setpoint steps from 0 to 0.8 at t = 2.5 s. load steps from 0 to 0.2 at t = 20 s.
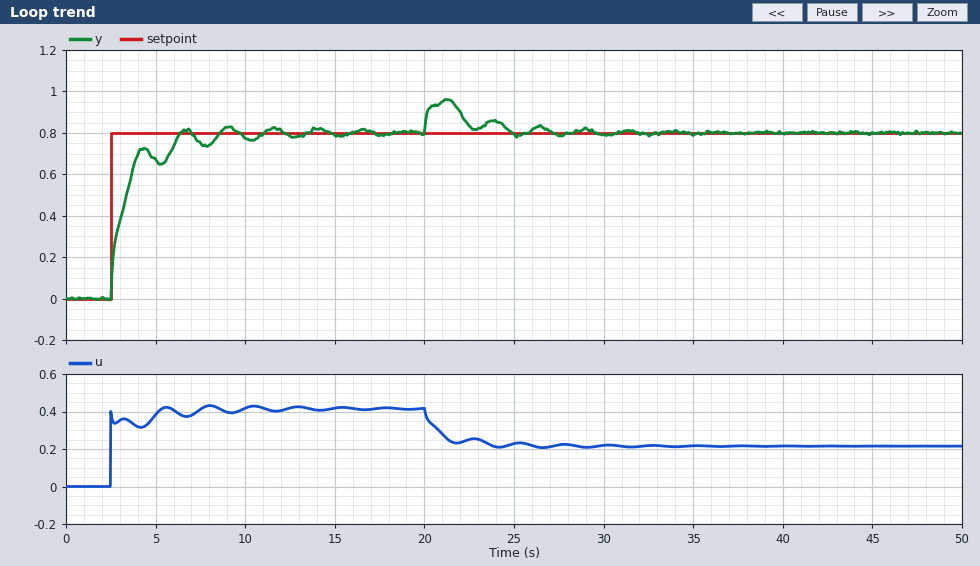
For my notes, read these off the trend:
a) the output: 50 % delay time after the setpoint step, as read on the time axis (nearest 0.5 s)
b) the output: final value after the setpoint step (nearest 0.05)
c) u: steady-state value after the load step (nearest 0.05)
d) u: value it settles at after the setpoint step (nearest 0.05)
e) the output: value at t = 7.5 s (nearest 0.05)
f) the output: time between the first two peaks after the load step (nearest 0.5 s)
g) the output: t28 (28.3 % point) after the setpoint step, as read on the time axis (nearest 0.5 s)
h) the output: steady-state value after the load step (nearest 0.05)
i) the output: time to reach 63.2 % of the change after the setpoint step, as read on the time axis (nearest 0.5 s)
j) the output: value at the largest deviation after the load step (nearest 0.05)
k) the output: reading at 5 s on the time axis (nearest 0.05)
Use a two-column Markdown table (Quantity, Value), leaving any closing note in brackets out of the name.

| Quantity | Value |
|---|---|
| the output: 50 % delay time after the setpoint step, as read on the time axis | 3.0 s |
| the output: final value after the setpoint step | 0.80 |
| u: steady-state value after the load step | 0.20 |
| u: value it settles at after the setpoint step | 0.40 |
| the output: value at t = 7.5 s | 0.75 |
| the output: time between the first two peaks after the load step | 2.5 s |
| the output: t28 (28.3 % point) after the setpoint step, as read on the time axis | 2.5 s |
| the output: steady-state value after the load step | 0.80 |
| the output: time to reach 63.2 % of the change after the setpoint step, as read on the time axis | 3.5 s |
| the output: value at the largest deviation after the load step | 0.95 |
| the output: reading at 5 s on the time axis | 0.65 |
